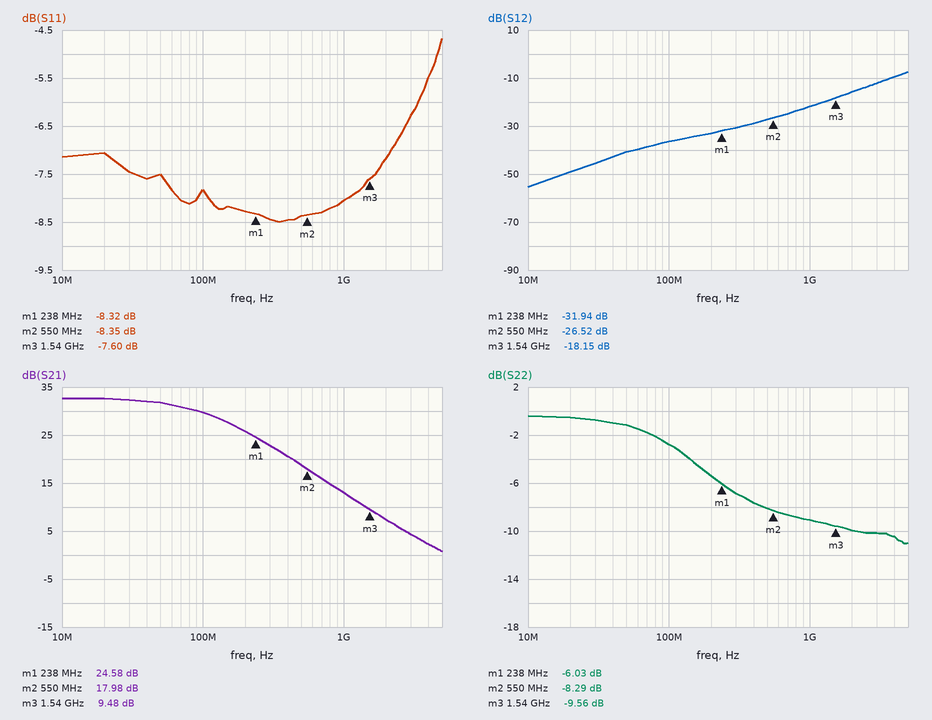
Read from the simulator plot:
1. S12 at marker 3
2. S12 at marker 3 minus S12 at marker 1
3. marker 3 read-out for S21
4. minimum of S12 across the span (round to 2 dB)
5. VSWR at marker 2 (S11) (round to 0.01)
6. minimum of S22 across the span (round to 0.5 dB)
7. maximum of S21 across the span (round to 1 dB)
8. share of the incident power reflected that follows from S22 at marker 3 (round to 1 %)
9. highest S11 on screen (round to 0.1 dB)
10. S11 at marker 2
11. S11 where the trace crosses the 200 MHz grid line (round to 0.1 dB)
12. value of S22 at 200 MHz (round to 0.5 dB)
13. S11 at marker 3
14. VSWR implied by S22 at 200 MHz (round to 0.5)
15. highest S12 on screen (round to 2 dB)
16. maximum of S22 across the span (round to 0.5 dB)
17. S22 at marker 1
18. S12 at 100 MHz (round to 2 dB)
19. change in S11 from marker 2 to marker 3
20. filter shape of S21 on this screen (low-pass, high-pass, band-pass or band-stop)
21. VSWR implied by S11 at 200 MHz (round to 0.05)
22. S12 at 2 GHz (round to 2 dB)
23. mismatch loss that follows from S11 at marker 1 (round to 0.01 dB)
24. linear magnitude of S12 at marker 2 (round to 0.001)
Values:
-18.15 dB
13.79 dB
9.48 dB
-56 dB
2.24
-11.0 dB
33 dB
11 %
-4.7 dB
-8.35 dB
-8.3 dB
-5.5 dB
-7.60 dB
3.5
-8 dB
-0.5 dB
-6.03 dB
-36 dB
0.75 dB
low-pass
2.25
-16 dB
0.69 dB
0.047
